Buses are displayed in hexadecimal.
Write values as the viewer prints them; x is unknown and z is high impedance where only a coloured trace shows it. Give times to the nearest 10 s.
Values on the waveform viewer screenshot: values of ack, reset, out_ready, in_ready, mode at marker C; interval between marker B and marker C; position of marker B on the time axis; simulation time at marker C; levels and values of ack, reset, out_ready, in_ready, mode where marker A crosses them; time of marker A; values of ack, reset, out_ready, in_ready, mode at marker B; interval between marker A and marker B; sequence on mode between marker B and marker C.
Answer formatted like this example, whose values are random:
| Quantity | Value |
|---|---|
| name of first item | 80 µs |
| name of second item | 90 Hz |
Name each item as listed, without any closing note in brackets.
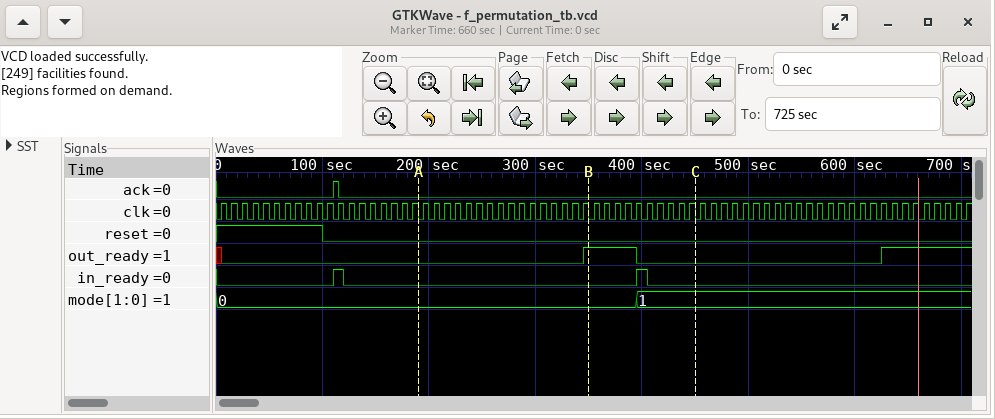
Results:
| Quantity | Value |
|---|---|
| values of ack, reset, out_ready, in_ready, mode at marker C | ack=0, reset=0, out_ready=0, in_ready=0, mode=1 |
| interval between marker B and marker C | 100 s |
| position of marker B on the time axis | 350 s |
| simulation time at marker C | 450 s |
| levels and values of ack, reset, out_ready, in_ready, mode where marker A crosses them | ack=0, reset=0, out_ready=0, in_ready=0, mode=0 |
| time of marker A | 190 s |
| values of ack, reset, out_ready, in_ready, mode at marker B | ack=0, reset=0, out_ready=1, in_ready=0, mode=0 |
| interval between marker A and marker B | 160 s |
| sequence on mode between marker B and marker C | 0, 1 |
